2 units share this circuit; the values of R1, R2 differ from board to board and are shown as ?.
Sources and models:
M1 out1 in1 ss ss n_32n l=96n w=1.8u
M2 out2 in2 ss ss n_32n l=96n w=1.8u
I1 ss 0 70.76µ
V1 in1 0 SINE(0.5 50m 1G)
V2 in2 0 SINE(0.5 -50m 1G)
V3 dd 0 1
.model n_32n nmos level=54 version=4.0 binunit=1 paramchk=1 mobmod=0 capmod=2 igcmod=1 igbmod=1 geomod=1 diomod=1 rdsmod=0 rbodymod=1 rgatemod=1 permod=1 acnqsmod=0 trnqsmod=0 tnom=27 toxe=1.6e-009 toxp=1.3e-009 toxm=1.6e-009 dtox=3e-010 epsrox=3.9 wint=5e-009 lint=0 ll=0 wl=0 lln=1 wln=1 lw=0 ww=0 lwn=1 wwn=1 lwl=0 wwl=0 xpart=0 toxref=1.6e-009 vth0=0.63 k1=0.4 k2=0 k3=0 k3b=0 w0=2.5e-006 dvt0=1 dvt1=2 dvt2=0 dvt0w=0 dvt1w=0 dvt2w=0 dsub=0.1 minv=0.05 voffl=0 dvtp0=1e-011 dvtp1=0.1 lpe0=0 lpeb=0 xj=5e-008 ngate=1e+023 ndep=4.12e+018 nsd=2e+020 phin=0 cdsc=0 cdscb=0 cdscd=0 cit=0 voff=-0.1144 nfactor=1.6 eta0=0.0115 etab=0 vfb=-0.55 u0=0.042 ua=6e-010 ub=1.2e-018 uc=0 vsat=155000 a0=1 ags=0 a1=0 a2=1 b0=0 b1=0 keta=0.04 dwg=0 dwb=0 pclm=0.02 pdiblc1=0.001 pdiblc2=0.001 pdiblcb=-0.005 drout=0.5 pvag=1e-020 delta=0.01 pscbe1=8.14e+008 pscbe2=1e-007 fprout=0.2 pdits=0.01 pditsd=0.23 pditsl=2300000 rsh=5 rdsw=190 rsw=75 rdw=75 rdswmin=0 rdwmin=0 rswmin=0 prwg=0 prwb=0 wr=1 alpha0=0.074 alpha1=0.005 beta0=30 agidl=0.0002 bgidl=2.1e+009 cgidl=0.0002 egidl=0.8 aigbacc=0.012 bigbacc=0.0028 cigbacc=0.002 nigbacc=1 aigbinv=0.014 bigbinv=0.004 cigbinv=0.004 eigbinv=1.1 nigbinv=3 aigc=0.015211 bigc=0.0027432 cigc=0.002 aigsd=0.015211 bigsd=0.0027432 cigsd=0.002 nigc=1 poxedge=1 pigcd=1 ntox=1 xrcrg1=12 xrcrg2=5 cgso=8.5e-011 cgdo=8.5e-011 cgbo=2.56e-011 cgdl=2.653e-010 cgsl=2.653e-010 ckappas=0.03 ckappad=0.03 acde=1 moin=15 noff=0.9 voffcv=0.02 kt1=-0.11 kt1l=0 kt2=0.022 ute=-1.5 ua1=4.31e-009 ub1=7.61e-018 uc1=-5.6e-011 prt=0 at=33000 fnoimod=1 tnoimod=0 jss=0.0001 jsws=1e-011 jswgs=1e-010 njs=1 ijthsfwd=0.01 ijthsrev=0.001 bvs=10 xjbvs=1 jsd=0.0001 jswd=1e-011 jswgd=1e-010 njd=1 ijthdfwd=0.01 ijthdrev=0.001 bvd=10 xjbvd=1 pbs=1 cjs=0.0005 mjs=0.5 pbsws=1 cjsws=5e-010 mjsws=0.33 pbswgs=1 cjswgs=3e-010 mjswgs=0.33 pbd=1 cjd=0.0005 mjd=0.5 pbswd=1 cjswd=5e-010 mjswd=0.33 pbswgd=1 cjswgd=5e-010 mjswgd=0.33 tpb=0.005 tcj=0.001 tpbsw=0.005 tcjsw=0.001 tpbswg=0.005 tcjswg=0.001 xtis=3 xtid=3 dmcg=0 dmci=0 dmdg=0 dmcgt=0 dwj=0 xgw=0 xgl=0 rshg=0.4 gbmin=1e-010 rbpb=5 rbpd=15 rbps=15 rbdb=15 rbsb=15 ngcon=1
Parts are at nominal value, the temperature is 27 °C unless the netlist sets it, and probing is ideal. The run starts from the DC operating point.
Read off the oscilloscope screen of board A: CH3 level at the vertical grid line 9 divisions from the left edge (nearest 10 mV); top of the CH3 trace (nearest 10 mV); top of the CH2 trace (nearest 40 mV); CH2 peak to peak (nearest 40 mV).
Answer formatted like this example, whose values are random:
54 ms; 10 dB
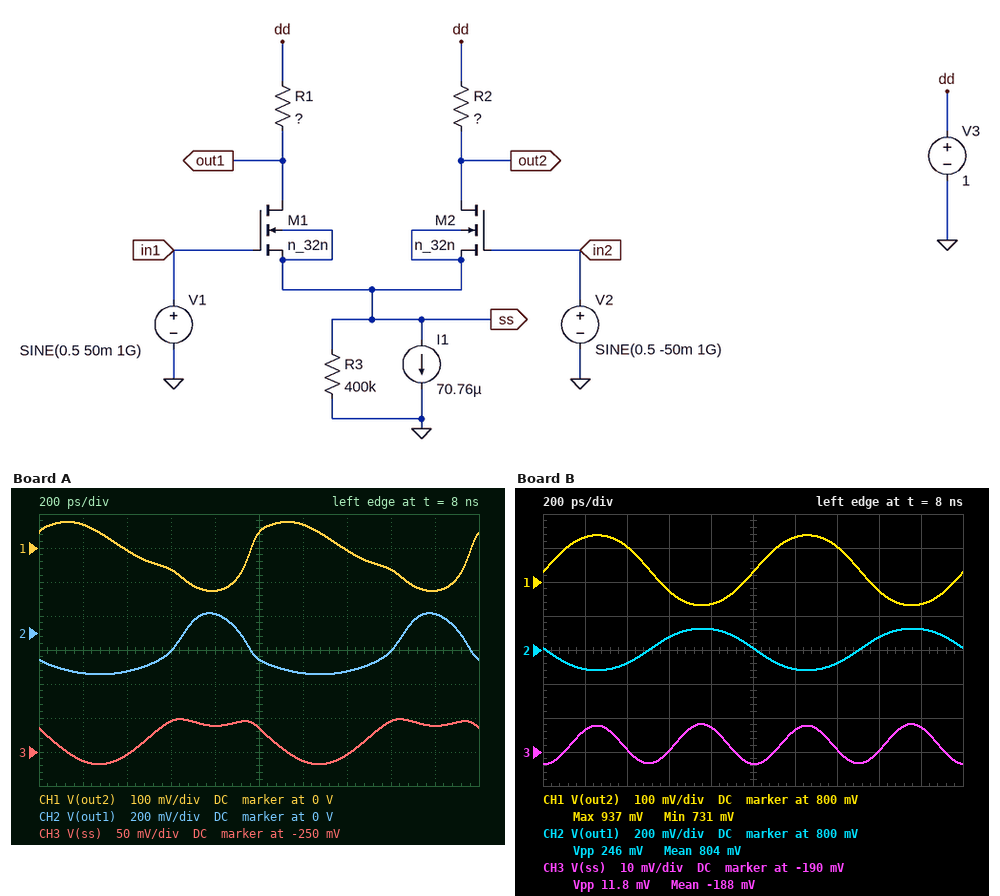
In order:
-210 mV; -200 mV; 120 mV; 360 mV
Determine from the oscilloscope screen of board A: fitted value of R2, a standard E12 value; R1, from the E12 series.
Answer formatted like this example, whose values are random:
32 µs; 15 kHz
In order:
22 kΩ; 47 kΩ
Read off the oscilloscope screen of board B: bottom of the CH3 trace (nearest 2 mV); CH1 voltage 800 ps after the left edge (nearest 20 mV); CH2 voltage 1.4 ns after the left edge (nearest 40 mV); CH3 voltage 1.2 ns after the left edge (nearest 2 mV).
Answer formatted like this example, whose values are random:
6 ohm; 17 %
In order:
-194 mV; 740 mV; 720 mV; -184 mV
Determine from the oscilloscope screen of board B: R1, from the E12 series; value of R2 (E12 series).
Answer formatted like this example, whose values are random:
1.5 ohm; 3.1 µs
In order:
5.6 kΩ; 4.7 kΩ
